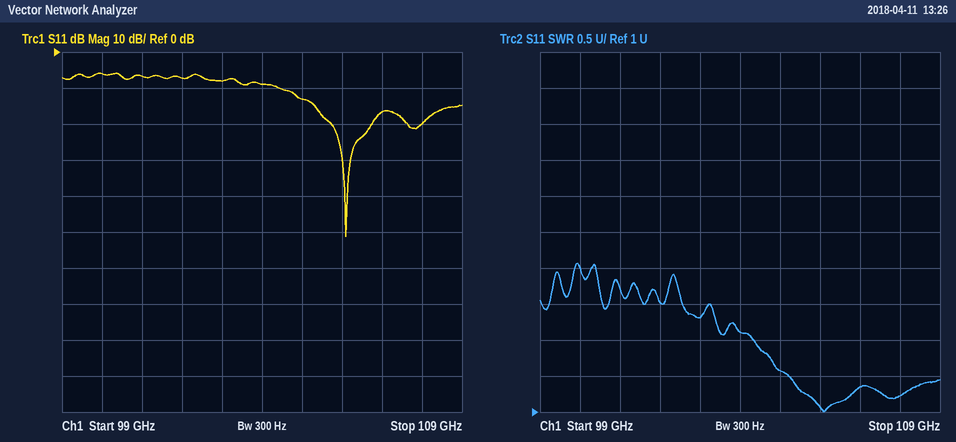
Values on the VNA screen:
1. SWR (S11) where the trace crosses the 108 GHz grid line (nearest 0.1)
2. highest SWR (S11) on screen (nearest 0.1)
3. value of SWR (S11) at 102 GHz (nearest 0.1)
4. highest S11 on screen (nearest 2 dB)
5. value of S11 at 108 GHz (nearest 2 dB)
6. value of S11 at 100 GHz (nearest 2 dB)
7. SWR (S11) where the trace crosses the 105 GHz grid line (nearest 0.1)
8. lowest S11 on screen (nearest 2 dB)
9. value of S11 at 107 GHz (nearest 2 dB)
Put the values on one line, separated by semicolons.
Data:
1.2; 3.1; 2.5; -6 dB; -20 dB; -6 dB; 1.6; -52 dB; -16 dB
